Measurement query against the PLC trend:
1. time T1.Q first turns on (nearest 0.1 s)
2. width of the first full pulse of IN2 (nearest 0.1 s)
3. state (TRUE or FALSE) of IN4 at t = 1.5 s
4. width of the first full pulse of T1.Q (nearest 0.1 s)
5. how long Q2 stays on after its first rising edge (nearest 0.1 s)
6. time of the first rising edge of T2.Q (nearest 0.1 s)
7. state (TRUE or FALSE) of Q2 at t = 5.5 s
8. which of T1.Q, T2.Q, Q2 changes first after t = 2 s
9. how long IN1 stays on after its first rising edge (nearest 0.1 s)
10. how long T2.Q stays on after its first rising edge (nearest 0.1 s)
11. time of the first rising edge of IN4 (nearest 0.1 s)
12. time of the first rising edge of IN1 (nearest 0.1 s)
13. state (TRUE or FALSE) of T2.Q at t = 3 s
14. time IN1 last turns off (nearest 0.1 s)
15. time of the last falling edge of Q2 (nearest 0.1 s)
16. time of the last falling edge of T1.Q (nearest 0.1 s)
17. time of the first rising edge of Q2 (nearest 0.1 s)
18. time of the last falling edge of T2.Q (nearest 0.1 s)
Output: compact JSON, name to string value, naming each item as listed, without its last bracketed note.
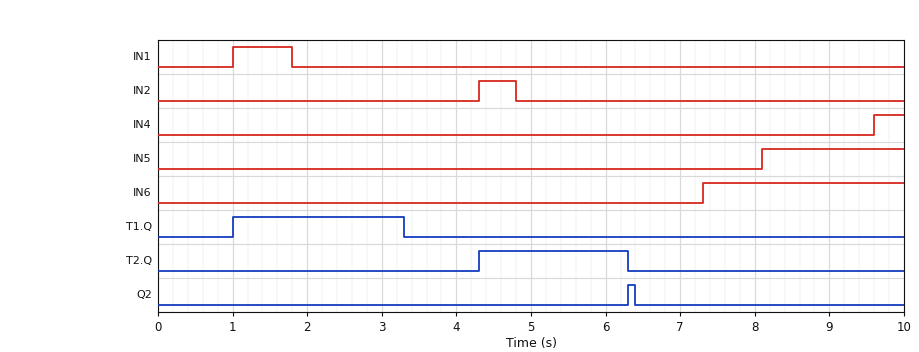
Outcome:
{"time T1.Q first turns on": "1.0 s", "width of the first full pulse of IN2": "0.5 s", "state (TRUE or FALSE) of IN4 at t = 1.5 s": "FALSE", "width of the first full pulse of T1.Q": "2.3 s", "how long Q2 stays on after its first rising edge": "0.1 s", "time of the first rising edge of T2.Q": "4.3 s", "state (TRUE or FALSE) of Q2 at t = 5.5 s": "FALSE", "which of T1.Q, T2.Q, Q2 changes first after t = 2 s": "T1.Q", "how long IN1 stays on after its first rising edge": "0.8 s", "how long T2.Q stays on after its first rising edge": "2.0 s", "time of the first rising edge of IN4": "9.6 s", "time of the first rising edge of IN1": "1.0 s", "state (TRUE or FALSE) of T2.Q at t = 3 s": "FALSE", "time IN1 last turns off": "1.8 s", "time of the last falling edge of Q2": "6.4 s", "time of the last falling edge of T1.Q": "3.3 s", "time of the first rising edge of Q2": "6.3 s", "time of the last falling edge of T2.Q": "6.3 s"}
